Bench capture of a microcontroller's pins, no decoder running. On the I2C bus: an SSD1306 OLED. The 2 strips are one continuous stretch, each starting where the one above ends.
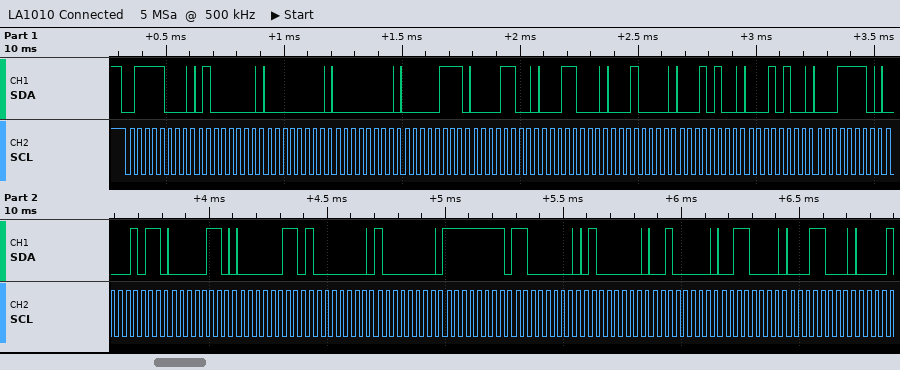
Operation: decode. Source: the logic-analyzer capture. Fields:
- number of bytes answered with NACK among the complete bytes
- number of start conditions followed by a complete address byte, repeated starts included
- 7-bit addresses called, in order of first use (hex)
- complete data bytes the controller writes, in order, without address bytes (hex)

0
1
0x3C
40 00 00 07 0C 18 10 14 14 1E 0B 06 03 80 80 FF C0 40 20 30 18
